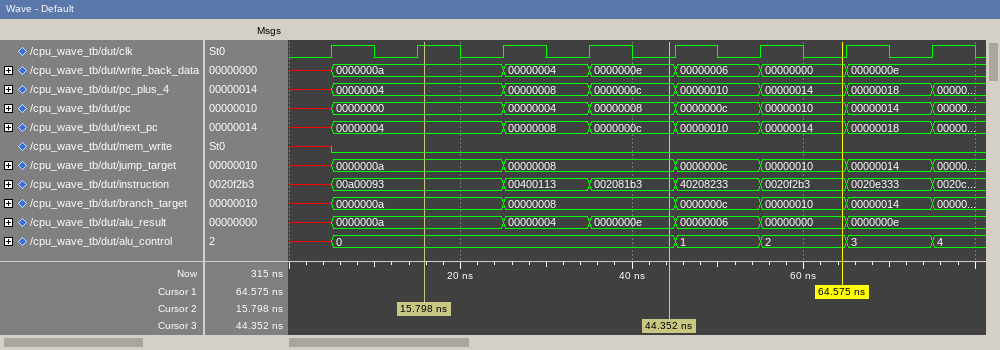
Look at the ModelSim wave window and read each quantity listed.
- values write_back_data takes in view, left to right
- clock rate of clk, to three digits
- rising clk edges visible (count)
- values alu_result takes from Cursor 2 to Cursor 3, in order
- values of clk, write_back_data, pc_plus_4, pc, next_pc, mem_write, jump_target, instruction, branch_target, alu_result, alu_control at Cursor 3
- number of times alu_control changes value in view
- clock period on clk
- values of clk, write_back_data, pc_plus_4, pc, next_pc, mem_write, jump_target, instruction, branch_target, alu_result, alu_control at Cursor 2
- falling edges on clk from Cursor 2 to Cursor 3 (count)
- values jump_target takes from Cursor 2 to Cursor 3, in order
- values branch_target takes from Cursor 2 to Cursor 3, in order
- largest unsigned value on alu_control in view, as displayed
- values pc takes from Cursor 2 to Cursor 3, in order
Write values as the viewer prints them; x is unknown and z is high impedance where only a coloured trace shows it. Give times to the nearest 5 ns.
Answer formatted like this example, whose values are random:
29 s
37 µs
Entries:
x, 0000000a, 00000004, 0000000e, 00000006, 00000000, 0000000e
100 MHz
8
0000000a, 00000004, 0000000e
clk=0, write_back_data=0000000e, pc_plus_4=0000000c, pc=00000008, next_pc=0000000c, mem_write=0, jump_target=00000008, instruction=002081b3, branch_target=00000008, alu_result=0000000e, alu_control=0
5
10 ns
clk=1, write_back_data=0000000a, pc_plus_4=00000004, pc=00000000, next_pc=00000004, mem_write=0, jump_target=0000000a, instruction=00a00093, branch_target=0000000a, alu_result=0000000a, alu_control=0
3
0000000a, 00000008
0000000a, 00000008
4
00000000, 00000004, 00000008
